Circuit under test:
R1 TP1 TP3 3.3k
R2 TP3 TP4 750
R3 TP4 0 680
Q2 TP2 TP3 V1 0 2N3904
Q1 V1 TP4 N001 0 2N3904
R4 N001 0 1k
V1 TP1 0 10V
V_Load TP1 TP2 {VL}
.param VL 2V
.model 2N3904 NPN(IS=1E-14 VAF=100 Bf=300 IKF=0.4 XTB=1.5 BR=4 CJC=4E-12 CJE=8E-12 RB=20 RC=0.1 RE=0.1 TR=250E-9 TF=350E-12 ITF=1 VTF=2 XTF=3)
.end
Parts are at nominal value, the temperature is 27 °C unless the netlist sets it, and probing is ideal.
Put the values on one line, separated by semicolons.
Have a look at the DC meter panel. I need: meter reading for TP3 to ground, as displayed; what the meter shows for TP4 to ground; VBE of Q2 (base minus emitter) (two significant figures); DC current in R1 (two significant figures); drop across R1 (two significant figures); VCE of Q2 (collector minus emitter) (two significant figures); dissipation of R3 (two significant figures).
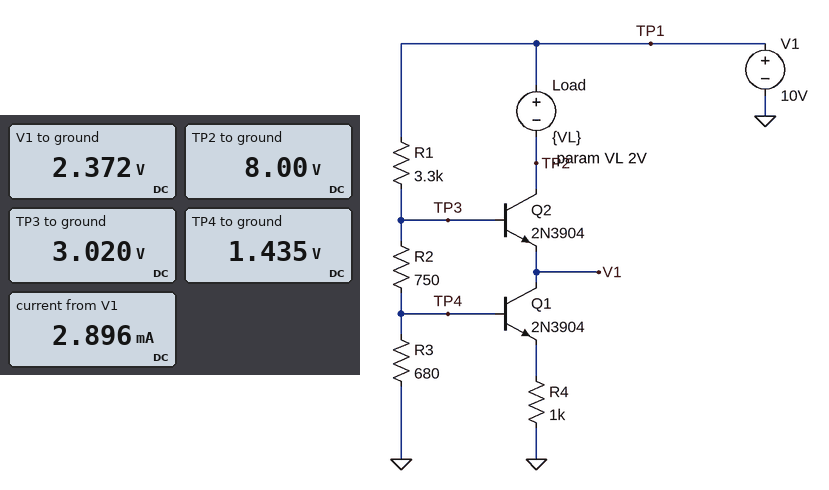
3.020 V; 1.435 V; 650 mV; 2.1 mA; 7.0 V; 5.6 V; 3.0 mW
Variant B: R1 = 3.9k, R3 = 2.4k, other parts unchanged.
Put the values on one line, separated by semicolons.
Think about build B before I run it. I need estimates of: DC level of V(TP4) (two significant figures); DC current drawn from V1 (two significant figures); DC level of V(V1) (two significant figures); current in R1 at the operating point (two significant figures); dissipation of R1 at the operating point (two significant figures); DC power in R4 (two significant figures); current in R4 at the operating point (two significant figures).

3.4 V; 4.1 mA; 3.8 V; 1.4 mA; 7.9 mW; 7.3 mW; 2.7 mA
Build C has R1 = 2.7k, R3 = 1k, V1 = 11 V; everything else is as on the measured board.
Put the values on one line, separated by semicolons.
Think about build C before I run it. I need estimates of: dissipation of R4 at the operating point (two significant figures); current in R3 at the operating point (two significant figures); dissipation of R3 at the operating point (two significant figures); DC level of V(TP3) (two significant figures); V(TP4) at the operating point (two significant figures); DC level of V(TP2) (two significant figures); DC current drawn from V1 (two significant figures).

3.2 mW; 2.5 mA; 6.1 mW; 4.3 V; 2.5 V; 9.0 V; 4.3 mA
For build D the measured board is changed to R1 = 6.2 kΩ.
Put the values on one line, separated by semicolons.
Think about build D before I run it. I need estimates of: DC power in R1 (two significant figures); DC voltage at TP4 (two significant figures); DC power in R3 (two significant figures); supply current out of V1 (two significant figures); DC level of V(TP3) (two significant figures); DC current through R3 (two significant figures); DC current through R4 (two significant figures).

11 mW; 890 mV; 1.2 mW; 1.6 mA; 1.9 V; 1.3 mA; 270 µA
